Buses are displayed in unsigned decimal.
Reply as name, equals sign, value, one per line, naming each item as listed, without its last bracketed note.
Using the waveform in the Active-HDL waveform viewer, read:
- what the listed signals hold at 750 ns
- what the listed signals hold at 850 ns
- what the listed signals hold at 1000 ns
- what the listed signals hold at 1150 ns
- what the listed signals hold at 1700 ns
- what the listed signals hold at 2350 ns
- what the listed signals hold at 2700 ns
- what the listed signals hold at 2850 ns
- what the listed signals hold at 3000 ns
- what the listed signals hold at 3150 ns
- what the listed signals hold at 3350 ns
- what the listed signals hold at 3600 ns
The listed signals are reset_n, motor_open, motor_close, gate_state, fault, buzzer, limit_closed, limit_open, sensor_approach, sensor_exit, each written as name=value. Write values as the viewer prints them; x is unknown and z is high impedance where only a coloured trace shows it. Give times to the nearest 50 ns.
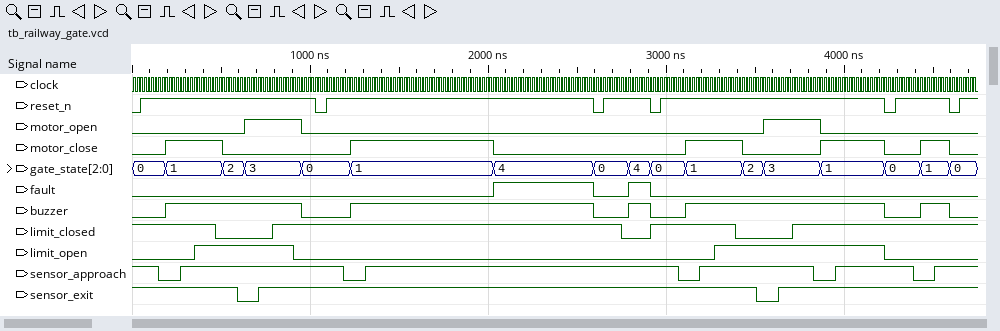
what the listed signals hold at 750 ns = reset_n=1, motor_open=1, motor_close=0, gate_state=3, fault=0, buzzer=1, limit_closed=0, limit_open=1, sensor_approach=1, sensor_exit=1
what the listed signals hold at 850 ns = reset_n=1, motor_open=1, motor_close=0, gate_state=3, fault=0, buzzer=1, limit_closed=1, limit_open=1, sensor_approach=1, sensor_exit=1
what the listed signals hold at 1000 ns = reset_n=1, motor_open=0, motor_close=0, gate_state=0, fault=0, buzzer=0, limit_closed=1, limit_open=0, sensor_approach=1, sensor_exit=1
what the listed signals hold at 1150 ns = reset_n=1, motor_open=0, motor_close=0, gate_state=0, fault=0, buzzer=0, limit_closed=1, limit_open=0, sensor_approach=1, sensor_exit=1
what the listed signals hold at 1700 ns = reset_n=1, motor_open=0, motor_close=1, gate_state=1, fault=0, buzzer=1, limit_closed=1, limit_open=0, sensor_approach=1, sensor_exit=1
what the listed signals hold at 2350 ns = reset_n=1, motor_open=0, motor_close=0, gate_state=4, fault=1, buzzer=1, limit_closed=1, limit_open=0, sensor_approach=1, sensor_exit=1
what the listed signals hold at 2700 ns = reset_n=1, motor_open=0, motor_close=0, gate_state=0, fault=0, buzzer=0, limit_closed=1, limit_open=0, sensor_approach=1, sensor_exit=1
what the listed signals hold at 2850 ns = reset_n=1, motor_open=0, motor_close=0, gate_state=4, fault=1, buzzer=1, limit_closed=0, limit_open=0, sensor_approach=1, sensor_exit=1
what the listed signals hold at 3000 ns = reset_n=1, motor_open=0, motor_close=0, gate_state=0, fault=0, buzzer=0, limit_closed=1, limit_open=0, sensor_approach=1, sensor_exit=1
what the listed signals hold at 3150 ns = reset_n=1, motor_open=0, motor_close=1, gate_state=1, fault=0, buzzer=1, limit_closed=1, limit_open=0, sensor_approach=0, sensor_exit=1
what the listed signals hold at 3350 ns = reset_n=1, motor_open=0, motor_close=1, gate_state=1, fault=0, buzzer=1, limit_closed=1, limit_open=1, sensor_approach=1, sensor_exit=1
what the listed signals hold at 3600 ns = reset_n=1, motor_open=1, motor_close=0, gate_state=3, fault=0, buzzer=1, limit_closed=0, limit_open=1, sensor_approach=1, sensor_exit=0
